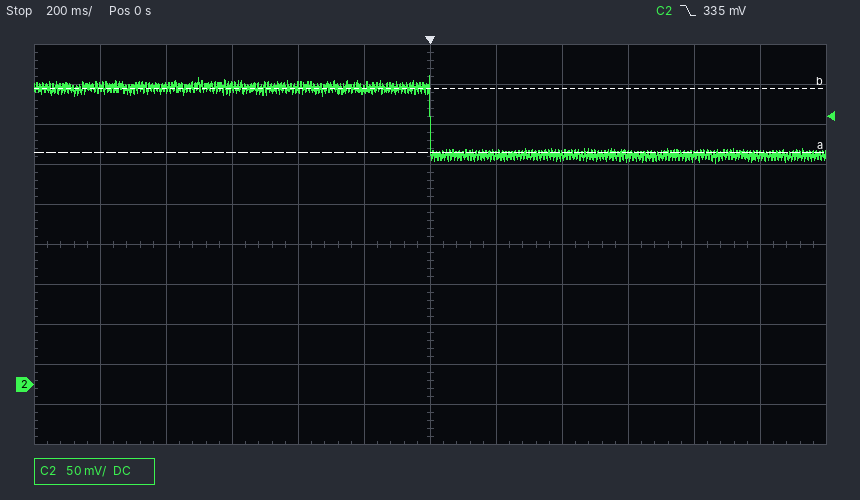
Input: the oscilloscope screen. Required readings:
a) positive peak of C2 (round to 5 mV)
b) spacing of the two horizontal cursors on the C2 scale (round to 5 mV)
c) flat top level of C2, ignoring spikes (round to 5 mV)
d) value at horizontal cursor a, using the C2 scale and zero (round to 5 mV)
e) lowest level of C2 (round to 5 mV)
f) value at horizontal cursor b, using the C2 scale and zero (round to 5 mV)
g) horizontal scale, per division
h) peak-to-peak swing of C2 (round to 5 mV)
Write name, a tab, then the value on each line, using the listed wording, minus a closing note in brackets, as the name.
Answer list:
positive peak of C2	385 mV
spacing of the two horizontal cursors on the C2 scale	80 mV
flat top level of C2, ignoring spikes	370 mV
value at horizontal cursor a, using the C2 scale and zero	290 mV
lowest level of C2	275 mV
value at horizontal cursor b, using the C2 scale and zero	370 mV
horizontal scale, per division	200 ms
peak-to-peak swing of C2	110 mV
